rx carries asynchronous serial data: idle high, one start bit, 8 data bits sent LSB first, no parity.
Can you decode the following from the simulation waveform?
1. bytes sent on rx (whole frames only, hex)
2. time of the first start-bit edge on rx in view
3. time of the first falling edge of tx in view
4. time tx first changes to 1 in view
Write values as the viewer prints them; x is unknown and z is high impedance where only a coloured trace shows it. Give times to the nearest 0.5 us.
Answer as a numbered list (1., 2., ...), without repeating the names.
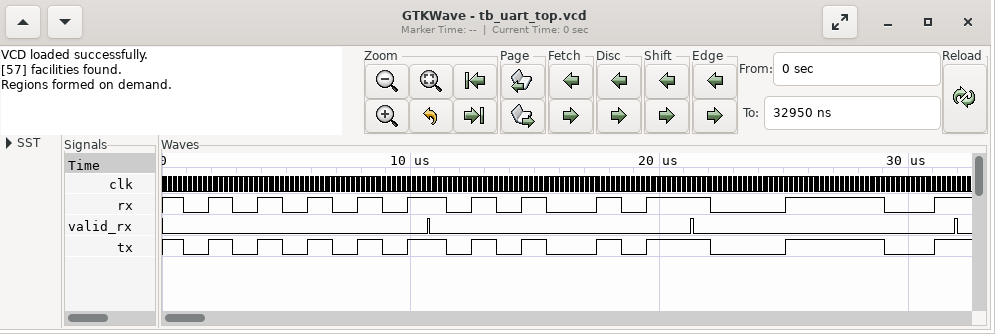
1. 55, A5, 3C
2. 1 us
3. 1 us
4. 2 us
